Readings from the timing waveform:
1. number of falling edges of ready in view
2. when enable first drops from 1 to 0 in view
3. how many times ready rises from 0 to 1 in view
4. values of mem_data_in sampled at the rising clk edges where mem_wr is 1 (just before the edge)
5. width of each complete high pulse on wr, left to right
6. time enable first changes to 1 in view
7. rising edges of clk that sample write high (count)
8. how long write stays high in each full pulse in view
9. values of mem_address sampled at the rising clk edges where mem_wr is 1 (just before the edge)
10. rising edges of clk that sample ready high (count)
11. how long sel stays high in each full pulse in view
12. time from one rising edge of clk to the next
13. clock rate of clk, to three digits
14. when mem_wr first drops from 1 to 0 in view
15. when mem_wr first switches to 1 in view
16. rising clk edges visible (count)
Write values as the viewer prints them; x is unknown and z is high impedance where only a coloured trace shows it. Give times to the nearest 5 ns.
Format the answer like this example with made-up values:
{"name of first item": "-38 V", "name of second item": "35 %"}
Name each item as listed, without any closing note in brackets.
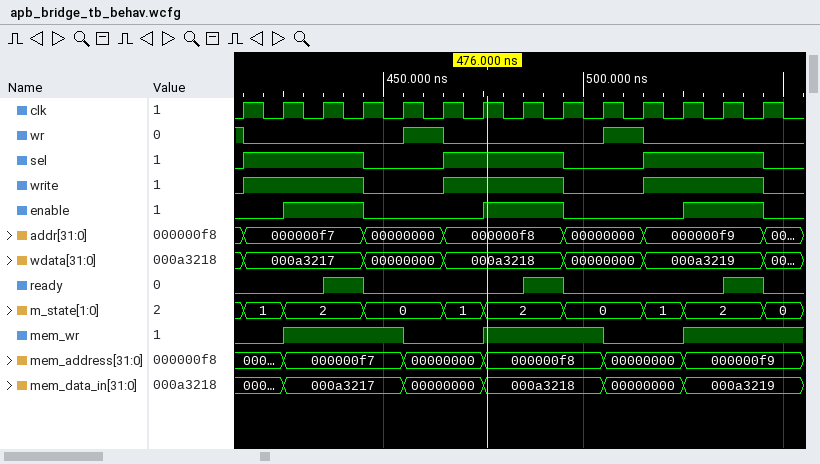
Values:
{"number of falling edges of ready in view": "3", "when enable first drops from 1 to 0 in view": "445 ns", "how many times ready rises from 0 to 1 in view": "3", "values of mem_data_in sampled at the rising clk edges where mem_wr is 1": "000a3217, 000a3217, 000a3217, 000a3218, 000a3218, 000a3218, 000a3219, 000a3219", "width of each complete high pulse on wr, left to right": "10 ns, 10 ns", "time enable first changes to 1 in view": "425 ns", "rising edges of clk that sample write high": "9", "how long write stays high in each full pulse in view": "30 ns, 30 ns, 30 ns", "values of mem_address sampled at the rising clk edges where mem_wr is 1": "000000f7, 000000f7, 000000f7, 000000f8, 000000f8, 000000f8, 000000f9, 000000f9", "rising edges of clk that sample ready high": "3", "how long sel stays high in each full pulse in view": "30 ns, 30 ns, 30 ns", "time from one rising edge of clk to the next": "10 ns", "clock rate of clk, to three digits": "100 MHz", "when mem_wr first drops from 1 to 0 in view": "455 ns", "when mem_wr first switches to 1 in view": "425 ns", "rising clk edges visible": "14"}
